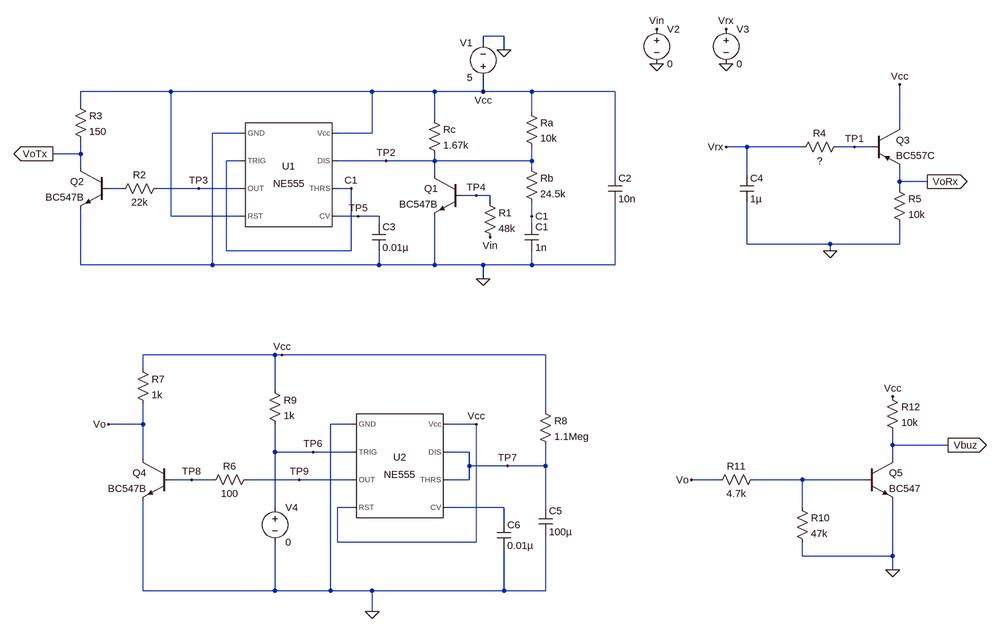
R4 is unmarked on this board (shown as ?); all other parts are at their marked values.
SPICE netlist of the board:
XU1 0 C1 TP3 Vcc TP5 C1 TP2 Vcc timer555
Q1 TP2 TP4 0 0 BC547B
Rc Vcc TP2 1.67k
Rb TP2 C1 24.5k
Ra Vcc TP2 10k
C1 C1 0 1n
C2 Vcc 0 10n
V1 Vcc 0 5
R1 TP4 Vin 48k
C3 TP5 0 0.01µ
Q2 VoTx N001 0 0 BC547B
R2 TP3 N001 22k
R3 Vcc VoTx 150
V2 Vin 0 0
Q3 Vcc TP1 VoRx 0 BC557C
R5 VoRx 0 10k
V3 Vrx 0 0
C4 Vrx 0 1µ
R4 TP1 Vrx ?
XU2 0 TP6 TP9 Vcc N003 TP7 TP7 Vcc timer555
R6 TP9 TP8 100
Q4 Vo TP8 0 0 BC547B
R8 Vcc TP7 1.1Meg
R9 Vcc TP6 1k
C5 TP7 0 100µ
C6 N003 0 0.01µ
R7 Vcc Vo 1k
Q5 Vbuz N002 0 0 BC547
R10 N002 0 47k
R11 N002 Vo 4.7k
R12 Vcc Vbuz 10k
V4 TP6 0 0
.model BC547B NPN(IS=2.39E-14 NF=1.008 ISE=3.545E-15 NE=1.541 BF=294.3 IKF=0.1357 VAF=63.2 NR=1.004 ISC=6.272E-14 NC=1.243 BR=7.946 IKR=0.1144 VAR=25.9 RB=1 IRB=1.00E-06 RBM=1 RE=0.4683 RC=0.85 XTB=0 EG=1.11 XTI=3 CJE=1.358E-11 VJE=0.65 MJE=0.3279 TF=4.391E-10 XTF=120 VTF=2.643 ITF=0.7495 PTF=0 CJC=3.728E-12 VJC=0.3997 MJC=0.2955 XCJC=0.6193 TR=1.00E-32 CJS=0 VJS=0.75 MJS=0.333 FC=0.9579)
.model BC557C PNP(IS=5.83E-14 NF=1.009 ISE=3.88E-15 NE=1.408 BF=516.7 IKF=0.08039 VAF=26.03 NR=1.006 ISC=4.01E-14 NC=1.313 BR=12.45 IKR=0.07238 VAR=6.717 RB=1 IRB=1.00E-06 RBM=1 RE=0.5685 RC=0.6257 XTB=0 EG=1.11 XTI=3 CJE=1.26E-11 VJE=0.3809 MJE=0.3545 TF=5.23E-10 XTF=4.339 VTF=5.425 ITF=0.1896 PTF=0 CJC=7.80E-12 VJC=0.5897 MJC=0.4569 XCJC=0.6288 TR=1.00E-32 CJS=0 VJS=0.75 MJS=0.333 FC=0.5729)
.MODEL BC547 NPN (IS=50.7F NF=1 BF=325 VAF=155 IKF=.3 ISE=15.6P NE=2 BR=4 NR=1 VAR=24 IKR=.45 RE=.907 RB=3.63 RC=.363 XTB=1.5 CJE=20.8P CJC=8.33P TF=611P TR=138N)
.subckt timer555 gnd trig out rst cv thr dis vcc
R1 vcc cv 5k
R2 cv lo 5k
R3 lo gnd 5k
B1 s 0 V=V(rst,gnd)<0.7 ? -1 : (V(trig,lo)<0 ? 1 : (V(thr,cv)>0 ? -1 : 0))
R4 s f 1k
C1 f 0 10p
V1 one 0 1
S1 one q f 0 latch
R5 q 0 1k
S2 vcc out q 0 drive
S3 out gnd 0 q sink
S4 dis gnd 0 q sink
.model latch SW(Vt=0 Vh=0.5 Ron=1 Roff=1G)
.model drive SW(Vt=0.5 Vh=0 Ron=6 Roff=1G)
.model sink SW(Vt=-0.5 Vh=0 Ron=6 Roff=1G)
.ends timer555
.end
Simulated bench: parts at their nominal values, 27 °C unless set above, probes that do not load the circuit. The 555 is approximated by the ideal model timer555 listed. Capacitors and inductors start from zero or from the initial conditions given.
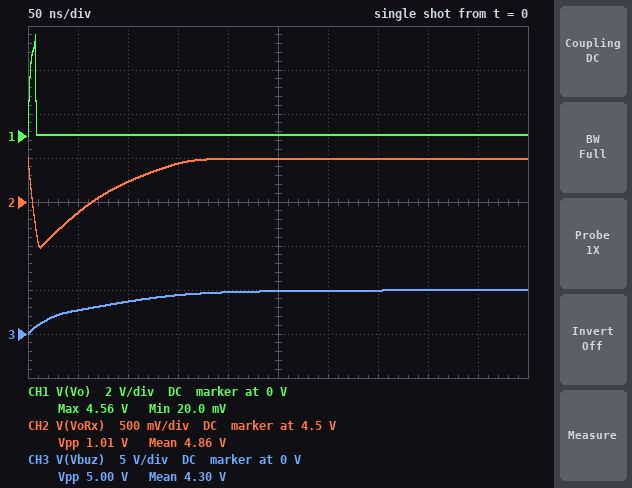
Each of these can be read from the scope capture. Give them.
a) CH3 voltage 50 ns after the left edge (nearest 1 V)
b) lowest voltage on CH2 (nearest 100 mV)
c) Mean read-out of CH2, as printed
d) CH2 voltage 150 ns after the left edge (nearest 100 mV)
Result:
3 V
4.0 V
4.86 V
4.9 V
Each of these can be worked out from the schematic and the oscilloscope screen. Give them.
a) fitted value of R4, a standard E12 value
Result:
27 kΩ
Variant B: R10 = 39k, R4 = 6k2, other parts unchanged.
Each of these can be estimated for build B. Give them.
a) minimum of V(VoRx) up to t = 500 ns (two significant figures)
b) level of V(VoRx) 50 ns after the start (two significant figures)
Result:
4.2 V
5.0 V
